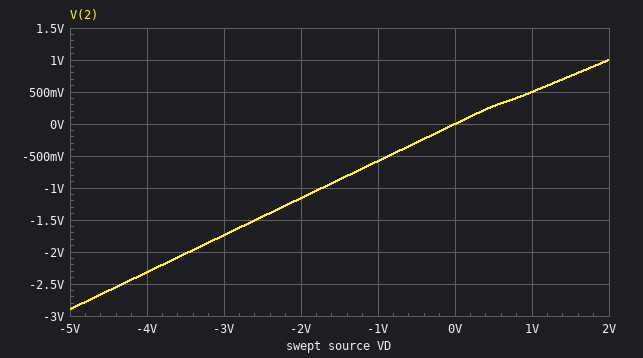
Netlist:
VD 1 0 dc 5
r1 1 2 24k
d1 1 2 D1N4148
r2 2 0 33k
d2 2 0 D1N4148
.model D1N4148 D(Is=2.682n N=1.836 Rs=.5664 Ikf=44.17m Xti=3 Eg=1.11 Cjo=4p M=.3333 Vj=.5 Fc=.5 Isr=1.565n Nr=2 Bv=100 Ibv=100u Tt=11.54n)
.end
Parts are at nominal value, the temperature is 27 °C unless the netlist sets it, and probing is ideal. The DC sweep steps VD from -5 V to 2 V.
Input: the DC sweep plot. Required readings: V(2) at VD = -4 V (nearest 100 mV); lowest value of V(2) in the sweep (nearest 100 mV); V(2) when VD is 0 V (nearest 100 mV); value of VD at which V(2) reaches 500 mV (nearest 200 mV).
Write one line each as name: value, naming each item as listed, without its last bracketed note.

V(2) at VD = -4 V: -2.3 V
lowest value of V(2) in the sweep: -2.9 V
V(2) when VD is 0 V: 0 V
value of VD at which V(2) reaches 500 mV: 1.0 V
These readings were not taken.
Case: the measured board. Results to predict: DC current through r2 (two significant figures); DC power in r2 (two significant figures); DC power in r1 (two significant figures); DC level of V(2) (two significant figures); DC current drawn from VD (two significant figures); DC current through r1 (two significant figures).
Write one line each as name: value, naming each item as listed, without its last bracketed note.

DC current through r2: 76 µA
DC power in r2: 190 µW
DC power in r1: 260 µW
DC level of V(2): 2.5 V
DC current drawn from VD: 2.4 A
DC current through r1: 100 µA
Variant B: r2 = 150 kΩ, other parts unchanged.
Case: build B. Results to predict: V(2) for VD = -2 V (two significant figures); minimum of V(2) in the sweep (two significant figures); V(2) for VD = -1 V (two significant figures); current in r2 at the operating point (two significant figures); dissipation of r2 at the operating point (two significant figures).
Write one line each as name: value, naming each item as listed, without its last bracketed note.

V(2) for VD = -2 V: -1.7 V
minimum of V(2) in the sweep: -4.3 V
V(2) for VD = -1 V: -860 mV
current in r2 at the operating point: 17 µA
dissipation of r2 at the operating point: 42 µW
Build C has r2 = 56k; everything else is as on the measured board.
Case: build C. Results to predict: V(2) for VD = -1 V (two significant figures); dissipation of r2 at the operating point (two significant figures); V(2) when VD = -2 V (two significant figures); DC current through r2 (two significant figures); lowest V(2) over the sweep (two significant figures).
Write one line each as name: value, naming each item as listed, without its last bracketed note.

V(2) for VD = -1 V: -700 mV
dissipation of r2 at the operating point: 110 µW
V(2) when VD = -2 V: -1.4 V
DC current through r2: 45 µA
lowest V(2) over the sweep: -3.5 V
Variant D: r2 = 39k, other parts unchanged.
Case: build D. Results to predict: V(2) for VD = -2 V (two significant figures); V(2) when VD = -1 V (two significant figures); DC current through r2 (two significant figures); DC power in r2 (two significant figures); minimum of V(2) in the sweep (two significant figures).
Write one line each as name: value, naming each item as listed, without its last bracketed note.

V(2) for VD = -2 V: -1.2 V
V(2) when VD = -1 V: -620 mV
DC current through r2: 64 µA
DC power in r2: 160 µW
minimum of V(2) in the sweep: -3.1 V
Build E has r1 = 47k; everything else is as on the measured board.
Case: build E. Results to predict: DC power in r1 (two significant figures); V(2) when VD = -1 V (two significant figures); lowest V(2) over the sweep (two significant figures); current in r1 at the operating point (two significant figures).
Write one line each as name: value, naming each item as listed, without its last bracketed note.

DC power in r1: 130 µW
V(2) when VD = -1 V: -410 mV
lowest V(2) over the sweep: -2.1 V
current in r1 at the operating point: 53 µA
